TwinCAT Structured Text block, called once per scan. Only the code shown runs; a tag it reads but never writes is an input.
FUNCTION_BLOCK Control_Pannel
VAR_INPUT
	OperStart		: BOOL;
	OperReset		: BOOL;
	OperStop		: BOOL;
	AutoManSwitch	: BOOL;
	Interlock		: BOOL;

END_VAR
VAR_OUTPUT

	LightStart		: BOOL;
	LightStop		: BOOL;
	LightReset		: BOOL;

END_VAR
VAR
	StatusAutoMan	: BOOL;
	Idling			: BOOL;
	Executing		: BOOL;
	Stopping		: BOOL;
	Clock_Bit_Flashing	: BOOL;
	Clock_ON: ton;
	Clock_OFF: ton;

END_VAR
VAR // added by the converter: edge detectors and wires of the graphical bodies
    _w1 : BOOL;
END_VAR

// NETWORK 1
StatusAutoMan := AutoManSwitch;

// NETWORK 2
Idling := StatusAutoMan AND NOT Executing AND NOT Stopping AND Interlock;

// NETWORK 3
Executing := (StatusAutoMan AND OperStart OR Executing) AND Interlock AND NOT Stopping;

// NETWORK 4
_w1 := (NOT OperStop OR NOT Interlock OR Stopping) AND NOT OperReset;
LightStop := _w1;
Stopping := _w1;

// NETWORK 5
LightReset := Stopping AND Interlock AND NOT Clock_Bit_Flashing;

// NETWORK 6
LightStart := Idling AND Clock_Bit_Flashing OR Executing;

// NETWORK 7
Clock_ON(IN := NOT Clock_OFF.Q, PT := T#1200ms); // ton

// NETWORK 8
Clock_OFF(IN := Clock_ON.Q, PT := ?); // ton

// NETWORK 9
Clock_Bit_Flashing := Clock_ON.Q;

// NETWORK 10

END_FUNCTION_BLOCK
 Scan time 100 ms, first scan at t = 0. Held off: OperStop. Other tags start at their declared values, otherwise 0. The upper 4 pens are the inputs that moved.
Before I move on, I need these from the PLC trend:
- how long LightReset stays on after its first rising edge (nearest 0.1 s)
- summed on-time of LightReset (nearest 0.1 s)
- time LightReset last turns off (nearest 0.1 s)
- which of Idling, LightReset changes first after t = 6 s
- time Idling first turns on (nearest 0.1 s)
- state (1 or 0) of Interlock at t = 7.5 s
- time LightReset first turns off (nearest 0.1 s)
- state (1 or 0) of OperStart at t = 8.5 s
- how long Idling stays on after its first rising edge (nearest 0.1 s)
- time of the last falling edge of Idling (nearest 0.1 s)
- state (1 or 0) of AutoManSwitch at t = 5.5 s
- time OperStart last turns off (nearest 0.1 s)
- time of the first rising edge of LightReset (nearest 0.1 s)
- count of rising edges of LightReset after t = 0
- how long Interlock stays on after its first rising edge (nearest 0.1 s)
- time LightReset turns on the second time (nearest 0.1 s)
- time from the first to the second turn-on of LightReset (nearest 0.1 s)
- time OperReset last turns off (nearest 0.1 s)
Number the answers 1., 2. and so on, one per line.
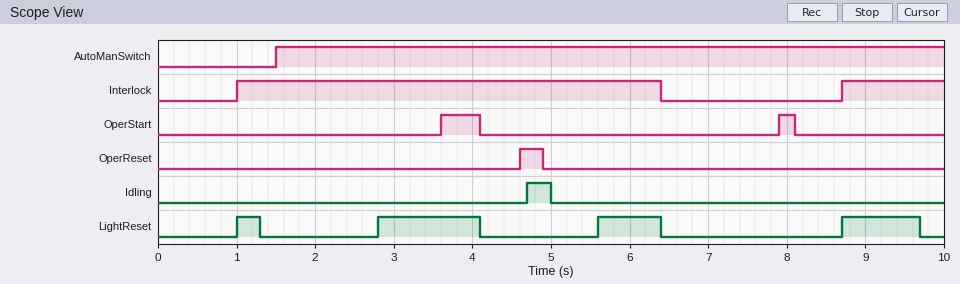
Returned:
1. 0.3 s
2. 3.4 s
3. 9.7 s
4. LightReset
5. 4.7 s
6. 0
7. 1.3 s
8. 0
9. 0.3 s
10. 5.0 s
11. 1
12. 8.1 s
13. 1.0 s
14. 4
15. 5.4 s
16. 2.8 s
17. 1.8 s
18. 4.9 s
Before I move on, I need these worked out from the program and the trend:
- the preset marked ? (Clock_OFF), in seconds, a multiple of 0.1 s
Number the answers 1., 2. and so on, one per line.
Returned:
1. 1.4 s
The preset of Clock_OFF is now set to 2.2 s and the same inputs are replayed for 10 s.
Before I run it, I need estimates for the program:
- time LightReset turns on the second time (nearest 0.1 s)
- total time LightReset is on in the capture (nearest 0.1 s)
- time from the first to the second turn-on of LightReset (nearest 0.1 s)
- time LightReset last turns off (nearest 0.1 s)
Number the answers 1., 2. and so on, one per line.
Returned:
1. 3.6 s
2. 1.3 s
3. 2.6 s
4. 4.6 s
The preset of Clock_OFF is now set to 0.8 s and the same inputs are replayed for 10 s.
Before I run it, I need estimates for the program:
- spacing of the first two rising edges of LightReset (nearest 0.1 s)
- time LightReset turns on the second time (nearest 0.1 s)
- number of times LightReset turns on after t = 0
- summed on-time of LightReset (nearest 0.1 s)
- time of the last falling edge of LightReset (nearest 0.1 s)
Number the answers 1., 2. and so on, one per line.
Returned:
1. 1.2 s
2. 2.2 s
3. 5
4. 3.8 s
5. 5.7 s
